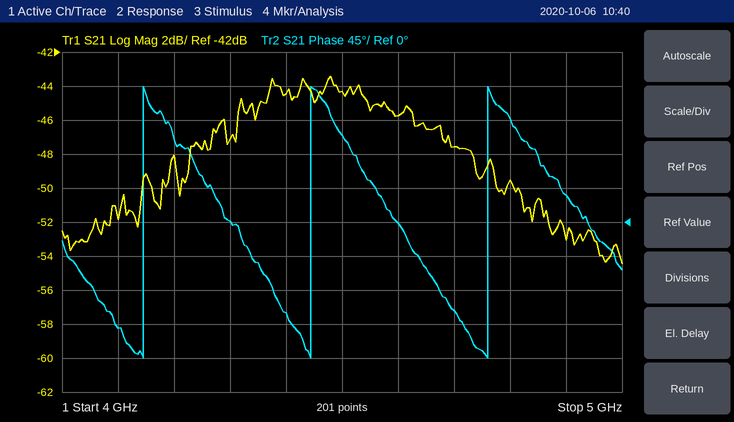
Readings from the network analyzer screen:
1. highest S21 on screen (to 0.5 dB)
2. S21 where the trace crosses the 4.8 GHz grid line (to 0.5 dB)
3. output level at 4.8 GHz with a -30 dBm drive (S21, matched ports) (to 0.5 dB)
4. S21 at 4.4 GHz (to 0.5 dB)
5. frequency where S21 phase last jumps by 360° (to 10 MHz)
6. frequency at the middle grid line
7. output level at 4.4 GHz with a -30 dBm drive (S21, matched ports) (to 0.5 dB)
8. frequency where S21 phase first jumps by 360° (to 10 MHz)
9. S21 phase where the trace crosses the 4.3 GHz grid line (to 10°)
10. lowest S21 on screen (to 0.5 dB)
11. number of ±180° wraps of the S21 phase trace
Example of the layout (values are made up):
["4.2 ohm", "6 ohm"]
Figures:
["-43.5 dB", "-49.5 dB", "-79.5 dBm", "-44.5 dB", "4.76 GHz", "4.5 GHz", "-74.5 dBm", "4.15 GHz", "0°", "-54.5 dB", "3"]
